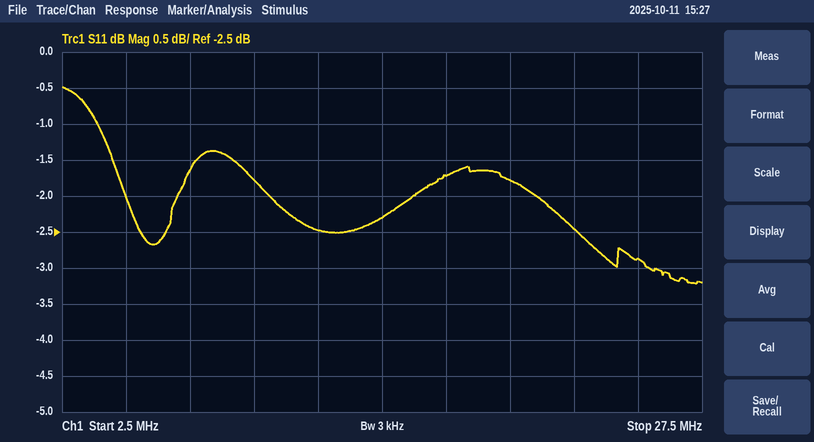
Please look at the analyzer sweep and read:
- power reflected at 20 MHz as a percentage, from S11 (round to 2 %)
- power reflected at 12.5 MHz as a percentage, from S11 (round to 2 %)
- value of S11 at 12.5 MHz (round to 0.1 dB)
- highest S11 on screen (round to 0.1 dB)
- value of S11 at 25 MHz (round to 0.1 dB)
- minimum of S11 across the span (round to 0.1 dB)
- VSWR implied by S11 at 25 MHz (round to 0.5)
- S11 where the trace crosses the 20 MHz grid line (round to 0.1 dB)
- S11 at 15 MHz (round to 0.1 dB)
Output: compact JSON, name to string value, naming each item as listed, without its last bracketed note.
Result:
{"power reflected at 20 MHz as a percentage, from S11": "66 %", "power reflected at 12.5 MHz as a percentage, from S11": "56 %", "value of S11 at 12.5 MHz": "-2.5 dB", "highest S11 on screen": "-0.5 dB", "value of S11 at 25 MHz": "-2.9 dB", "minimum of S11 across the span": "-3.2 dB", "VSWR implied by S11 at 25 MHz": "6.0", "S11 where the trace crosses the 20 MHz grid line": "-1.8 dB", "S11 at 15 MHz": "-2.3 dB"}
